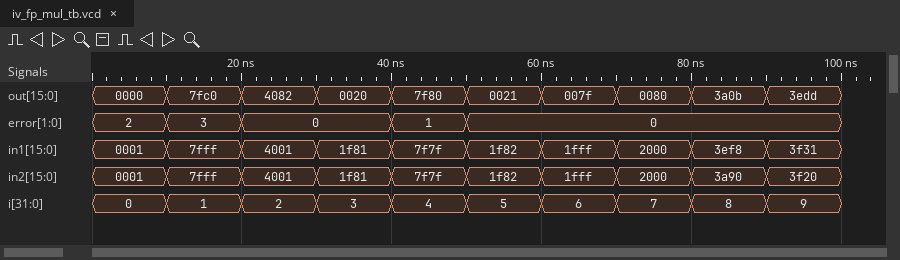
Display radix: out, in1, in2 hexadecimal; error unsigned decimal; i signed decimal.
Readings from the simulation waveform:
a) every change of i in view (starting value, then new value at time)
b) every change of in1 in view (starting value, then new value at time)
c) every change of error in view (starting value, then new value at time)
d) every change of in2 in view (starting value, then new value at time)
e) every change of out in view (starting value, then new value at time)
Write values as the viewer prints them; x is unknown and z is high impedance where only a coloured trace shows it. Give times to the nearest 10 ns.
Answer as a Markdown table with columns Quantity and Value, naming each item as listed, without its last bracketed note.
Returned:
| Quantity | Value |
|---|---|
| every change of i in view | 0, 1 at 10 ns, 2 at 20 ns, 3 at 30 ns, 4 at 40 ns, 5 at 50 ns, 6 at 60 ns, 7 at 70 ns, 8 at 80 ns, 9 at 90 ns |
| every change of in1 in view | 0001, 7fff at 10 ns, 4001 at 20 ns, 1f81 at 30 ns, 7f7f at 40 ns, 1f82 at 50 ns, 1fff at 60 ns, 2000 at 70 ns, 3ef8 at 80 ns, 3f31 at 90 ns |
| every change of error in view | 2, 3 at 10 ns, 0 at 20 ns, 1 at 40 ns, 0 at 50 ns |
| every change of in2 in view | 0001, 7fff at 10 ns, 4001 at 20 ns, 1f81 at 30 ns, 7f7f at 40 ns, 1f82 at 50 ns, 1fff at 60 ns, 2000 at 70 ns, 3a90 at 80 ns, 3f20 at 90 ns |
| every change of out in view | 0000, 7fc0 at 10 ns, 4082 at 20 ns, 0020 at 30 ns, 7f80 at 40 ns, 0021 at 50 ns, 007f at 60 ns, 0080 at 70 ns, 3a0b at 80 ns, 3edd at 90 ns |
